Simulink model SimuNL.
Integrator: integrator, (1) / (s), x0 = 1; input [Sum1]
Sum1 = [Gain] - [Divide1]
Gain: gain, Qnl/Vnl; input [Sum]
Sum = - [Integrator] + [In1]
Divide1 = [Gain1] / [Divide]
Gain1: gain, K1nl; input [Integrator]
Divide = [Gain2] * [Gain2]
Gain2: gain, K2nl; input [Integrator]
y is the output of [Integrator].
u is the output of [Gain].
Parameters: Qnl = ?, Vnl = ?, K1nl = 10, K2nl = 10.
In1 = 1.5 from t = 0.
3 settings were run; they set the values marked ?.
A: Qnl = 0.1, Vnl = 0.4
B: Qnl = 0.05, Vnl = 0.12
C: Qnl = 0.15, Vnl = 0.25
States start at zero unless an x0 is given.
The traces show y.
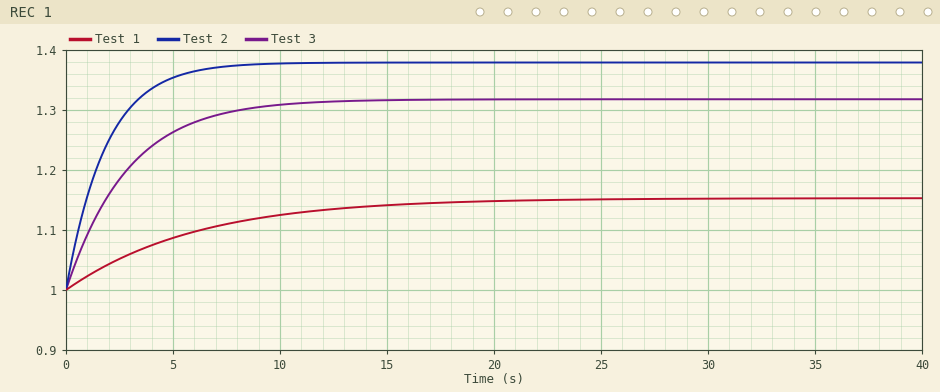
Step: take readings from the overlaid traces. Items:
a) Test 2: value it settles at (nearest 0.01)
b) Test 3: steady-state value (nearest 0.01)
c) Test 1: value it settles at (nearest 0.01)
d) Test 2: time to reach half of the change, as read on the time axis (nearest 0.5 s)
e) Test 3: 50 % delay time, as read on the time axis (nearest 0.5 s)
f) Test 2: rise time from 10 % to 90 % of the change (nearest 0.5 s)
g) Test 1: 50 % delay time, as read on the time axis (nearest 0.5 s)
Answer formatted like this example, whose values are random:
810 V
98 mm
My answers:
1.38
1.32
1.15
1.5 s
2.0 s
4.0 s
4.0 s
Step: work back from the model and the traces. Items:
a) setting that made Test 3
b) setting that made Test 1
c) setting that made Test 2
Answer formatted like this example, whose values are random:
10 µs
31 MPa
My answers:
B
A
C
